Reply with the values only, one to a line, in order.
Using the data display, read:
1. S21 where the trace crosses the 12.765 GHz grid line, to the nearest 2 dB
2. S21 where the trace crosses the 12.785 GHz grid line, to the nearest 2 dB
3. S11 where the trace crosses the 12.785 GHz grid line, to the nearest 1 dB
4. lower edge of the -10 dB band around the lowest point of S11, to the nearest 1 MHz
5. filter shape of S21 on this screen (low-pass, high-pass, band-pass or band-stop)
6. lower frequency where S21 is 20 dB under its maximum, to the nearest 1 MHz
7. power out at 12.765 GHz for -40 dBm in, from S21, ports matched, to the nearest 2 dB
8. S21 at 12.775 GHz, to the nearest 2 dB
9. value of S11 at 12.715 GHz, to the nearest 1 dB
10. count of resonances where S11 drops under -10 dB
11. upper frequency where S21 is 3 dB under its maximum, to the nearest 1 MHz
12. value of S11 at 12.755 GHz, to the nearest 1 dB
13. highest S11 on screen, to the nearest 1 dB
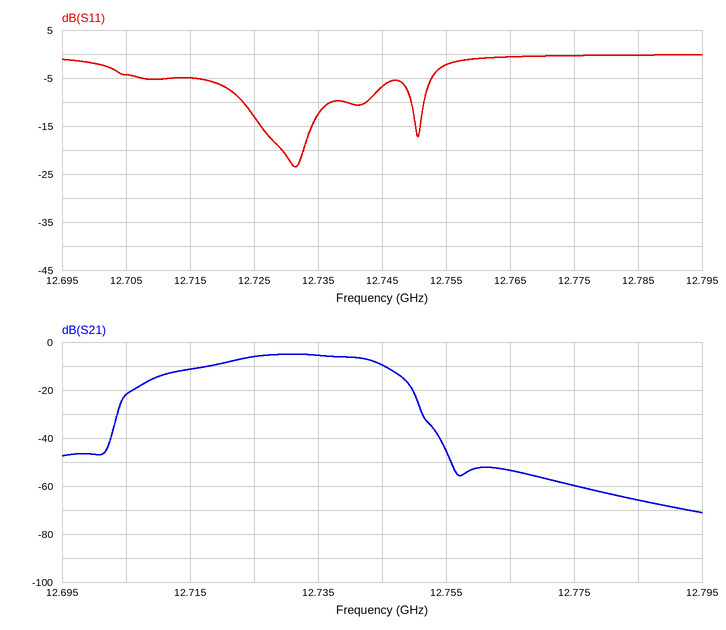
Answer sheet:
-54 dB
-66 dB
0 dB
12.723 GHz
band-pass
12.704 GHz
-94 dBm
-60 dB
-5 dB
2
12.744 GHz
-2 dB
0 dB
